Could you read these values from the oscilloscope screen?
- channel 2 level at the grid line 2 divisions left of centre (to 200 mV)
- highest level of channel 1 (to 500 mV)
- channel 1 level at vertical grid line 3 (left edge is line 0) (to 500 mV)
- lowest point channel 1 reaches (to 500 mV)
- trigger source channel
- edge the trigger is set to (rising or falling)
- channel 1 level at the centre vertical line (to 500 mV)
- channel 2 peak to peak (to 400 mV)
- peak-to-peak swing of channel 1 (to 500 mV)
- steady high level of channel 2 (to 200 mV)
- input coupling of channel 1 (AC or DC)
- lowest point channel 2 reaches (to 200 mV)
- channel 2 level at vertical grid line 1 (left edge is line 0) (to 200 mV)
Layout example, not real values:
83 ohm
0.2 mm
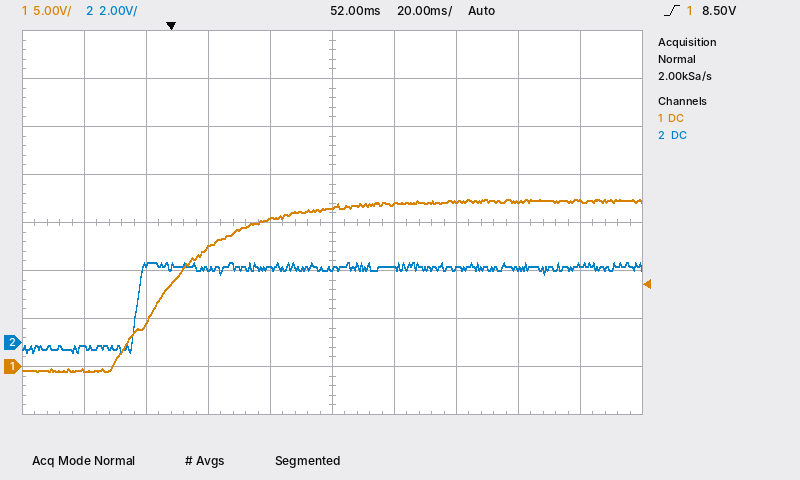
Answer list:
3.0 V
17.5 V
12.5 V
-500 mV
channel 1
rising
16.5 V
3.6 V
18.0 V
3.2 V
DC
-400 mV
-200 mV
